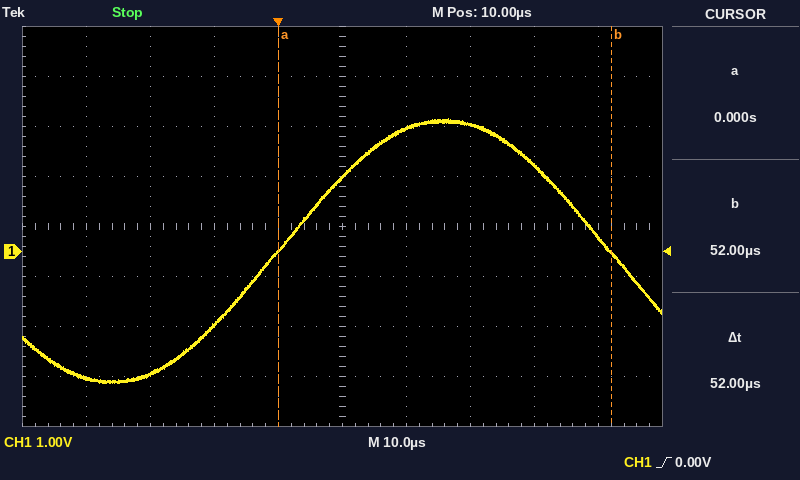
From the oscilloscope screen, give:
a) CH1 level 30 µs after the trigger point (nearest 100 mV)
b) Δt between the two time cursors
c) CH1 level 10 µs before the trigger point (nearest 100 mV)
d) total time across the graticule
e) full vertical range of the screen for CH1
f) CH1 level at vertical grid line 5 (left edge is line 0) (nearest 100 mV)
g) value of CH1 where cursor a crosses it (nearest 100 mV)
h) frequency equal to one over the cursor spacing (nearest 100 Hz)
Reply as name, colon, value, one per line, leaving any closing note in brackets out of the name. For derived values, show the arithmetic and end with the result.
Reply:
CH1 level 30 µs after the trigger point: 2.5 V
Δt between the two time cursors: 52 µs
CH1 level 10 µs before the trigger point: -1.5 V
total time across the graticule: 100 µs
full vertical range of the screen for CH1: 8 V
CH1 level at vertical grid line 5 (left edge is line 0): 1.5 V
value of CH1 where cursor a crosses it: 0.0 V
frequency equal to one over the cursor spacing: 1 / 52 µs ≈ 19.2 kHz
